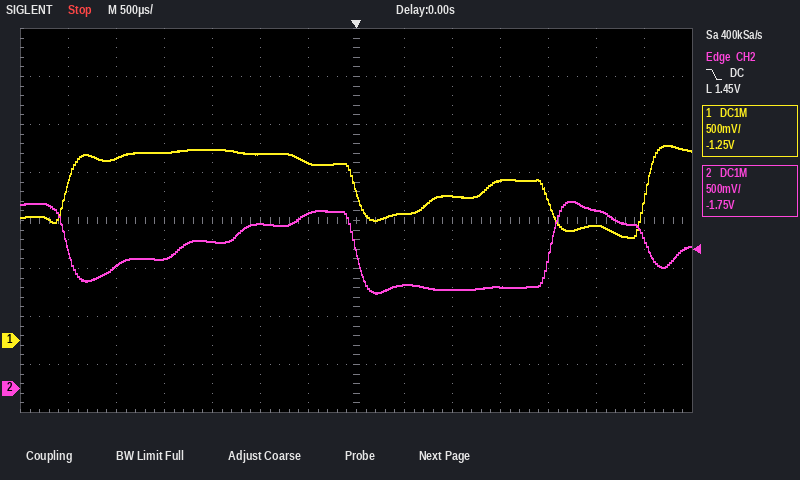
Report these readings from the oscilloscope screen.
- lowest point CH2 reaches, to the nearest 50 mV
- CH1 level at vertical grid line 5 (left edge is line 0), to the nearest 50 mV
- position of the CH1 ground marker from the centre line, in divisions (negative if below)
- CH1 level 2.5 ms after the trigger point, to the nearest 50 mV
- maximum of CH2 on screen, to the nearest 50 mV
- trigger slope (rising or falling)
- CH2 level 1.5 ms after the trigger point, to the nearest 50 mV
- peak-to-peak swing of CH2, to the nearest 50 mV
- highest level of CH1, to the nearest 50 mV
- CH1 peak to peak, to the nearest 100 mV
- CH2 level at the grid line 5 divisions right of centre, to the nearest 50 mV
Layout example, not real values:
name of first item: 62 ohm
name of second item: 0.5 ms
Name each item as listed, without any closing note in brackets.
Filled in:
lowest point CH2 reaches, to the nearest 50 mV: 1.00 V
CH1 level at vertical grid line 5 (left edge is line 0), to the nearest 50 mV: 1.95 V
position of the CH1 ground marker from the centre line, in divisions: -2.5 div
CH1 level 2.5 ms after the trigger point, to the nearest 50 mV: 1.20 V
maximum of CH2 on screen, to the nearest 50 mV: 1.95 V
trigger slope: falling
CH2 level 1.5 ms after the trigger point, to the nearest 50 mV: 1.05 V
peak-to-peak swing of CH2, to the nearest 50 mV: 950 mV
highest level of CH1, to the nearest 50 mV: 2.05 V
CH1 peak to peak, to the nearest 100 mV: 1.00 V
CH2 level at the grid line 5 divisions right of centre, to the nearest 50 mV: 1.85 V
